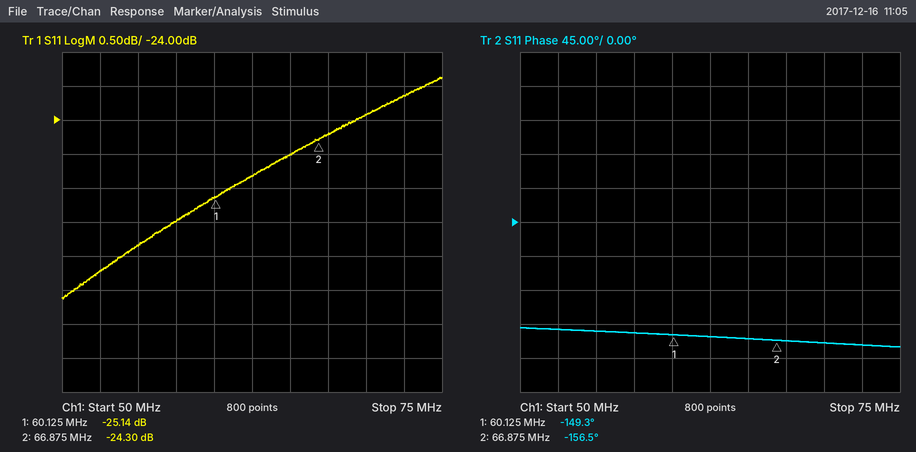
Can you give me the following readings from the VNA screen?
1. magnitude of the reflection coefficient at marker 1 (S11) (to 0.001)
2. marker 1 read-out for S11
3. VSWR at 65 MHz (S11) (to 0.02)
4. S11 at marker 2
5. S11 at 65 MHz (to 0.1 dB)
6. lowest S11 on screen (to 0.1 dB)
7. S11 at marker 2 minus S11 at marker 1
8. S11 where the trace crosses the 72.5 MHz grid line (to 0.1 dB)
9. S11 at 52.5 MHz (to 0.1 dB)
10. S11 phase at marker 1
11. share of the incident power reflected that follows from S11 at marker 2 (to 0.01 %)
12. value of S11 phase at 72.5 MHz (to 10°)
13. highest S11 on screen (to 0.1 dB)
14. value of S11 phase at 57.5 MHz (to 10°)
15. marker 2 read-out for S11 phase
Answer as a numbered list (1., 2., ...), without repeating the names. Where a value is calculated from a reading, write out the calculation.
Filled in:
1. 10^(-25.14/20) ≈ 0.055
2. -25.14 dB
3. |Γ| = 10^(-24.5/20) = 0.0596; VSWR = (1 + 0.0596)/(1 − 0.0596) ≈ 1.13, so 1.12 to the nearest 0.02
4. -24.30 dB
5. -24.5 dB
6. -26.6 dB
7. -24.3 − (-25.14) = 0.84 dB
8. -23.6 dB
9. -26.2 dB
10. -149.3°
11. 10^(-24.3/10) ≈ 0.37 %
12. -160°
13. -23.4 dB
14. -150°
15. -156.5°
